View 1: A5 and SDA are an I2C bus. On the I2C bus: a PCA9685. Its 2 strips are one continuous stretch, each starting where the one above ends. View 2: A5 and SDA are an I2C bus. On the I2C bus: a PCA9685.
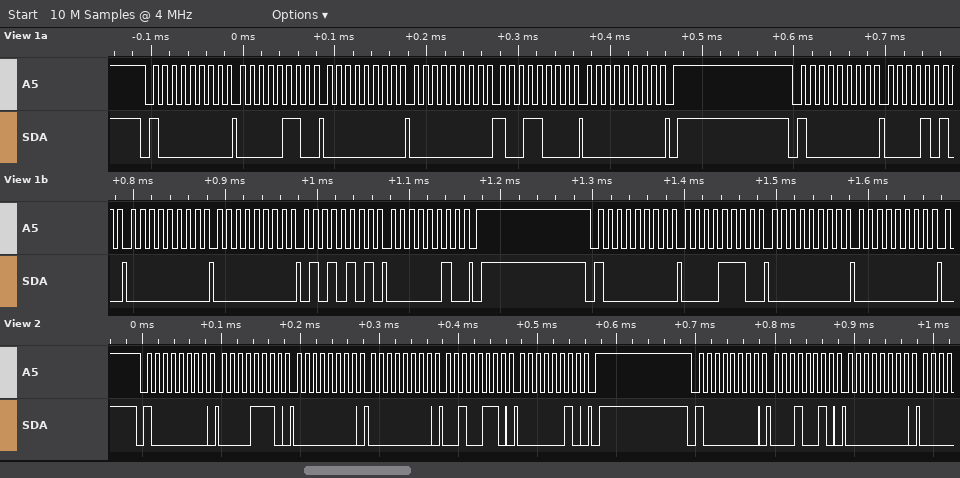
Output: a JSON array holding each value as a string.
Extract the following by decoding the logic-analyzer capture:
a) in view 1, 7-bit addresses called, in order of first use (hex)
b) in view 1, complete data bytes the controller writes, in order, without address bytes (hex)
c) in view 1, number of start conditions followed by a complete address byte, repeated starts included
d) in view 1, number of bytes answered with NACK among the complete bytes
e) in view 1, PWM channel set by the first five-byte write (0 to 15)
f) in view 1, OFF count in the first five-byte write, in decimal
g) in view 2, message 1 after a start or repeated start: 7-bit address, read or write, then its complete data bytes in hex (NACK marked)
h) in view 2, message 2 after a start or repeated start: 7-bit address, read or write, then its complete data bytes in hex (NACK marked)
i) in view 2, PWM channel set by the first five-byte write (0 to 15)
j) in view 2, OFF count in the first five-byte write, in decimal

["0x40", "06 00 00 98 00 0A 00 00 55 02 0E 00 00", "3", "0", "0", "152", "0x40 write: 0E 00 00 26 02", "0x40 write: 12 00", "2", "550"]
